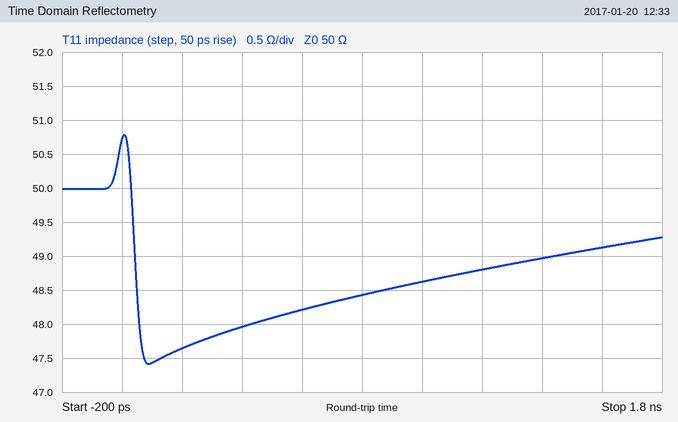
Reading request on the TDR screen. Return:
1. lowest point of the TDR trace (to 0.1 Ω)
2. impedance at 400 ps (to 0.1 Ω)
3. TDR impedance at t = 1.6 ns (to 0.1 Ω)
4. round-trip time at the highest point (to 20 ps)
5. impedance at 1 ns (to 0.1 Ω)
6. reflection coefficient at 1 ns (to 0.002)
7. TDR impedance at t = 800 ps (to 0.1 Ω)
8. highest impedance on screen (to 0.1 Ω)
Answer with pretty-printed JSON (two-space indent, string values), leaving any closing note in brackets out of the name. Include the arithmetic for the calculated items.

{
  "lowest point of the TDR trace": "47.4 Ω",
  "impedance at 400 ps": "48.0 Ω",
  "TDR impedance at t = 1.6 ns": "49.1 Ω",
  "round-trip time at the highest point": "0 ps",
  "impedance at 1 ns": "48.6 Ω",
  "reflection coefficient at 1 ns": "(48.6 − 50)/(48.6 + 50) ≈ -0.014",
  "TDR impedance at t = 800 ps": "48.4 Ω",
  "highest impedance on screen": "50.8 Ω"
}
